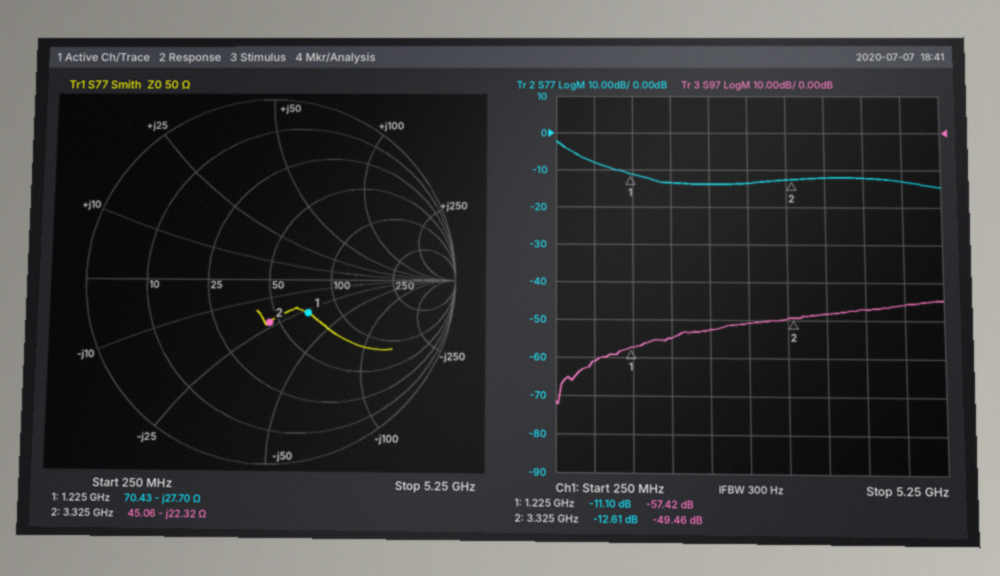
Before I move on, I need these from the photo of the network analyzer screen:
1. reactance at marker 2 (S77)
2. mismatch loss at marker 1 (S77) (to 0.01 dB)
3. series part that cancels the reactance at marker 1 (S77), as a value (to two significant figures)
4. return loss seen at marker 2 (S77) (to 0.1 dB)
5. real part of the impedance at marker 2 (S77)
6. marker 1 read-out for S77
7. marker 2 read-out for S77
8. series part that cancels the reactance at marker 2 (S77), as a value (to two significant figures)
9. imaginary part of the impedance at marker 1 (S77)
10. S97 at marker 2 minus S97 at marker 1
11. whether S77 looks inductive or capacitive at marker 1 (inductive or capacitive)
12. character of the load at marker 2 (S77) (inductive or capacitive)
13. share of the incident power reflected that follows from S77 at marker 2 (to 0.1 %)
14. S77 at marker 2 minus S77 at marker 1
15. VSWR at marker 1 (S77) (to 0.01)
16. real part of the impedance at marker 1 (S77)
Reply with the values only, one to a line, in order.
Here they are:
-22.32 Ω
0.35 dB
3.6 nH
12.6 dB
45.06 Ω
-11.10 dB
-12.61 dB
1.1 nH
-27.70 Ω
7.96 dB
capacitive
capacitive
5.5 %
-1.51 dB
1.77
70.43 Ω
